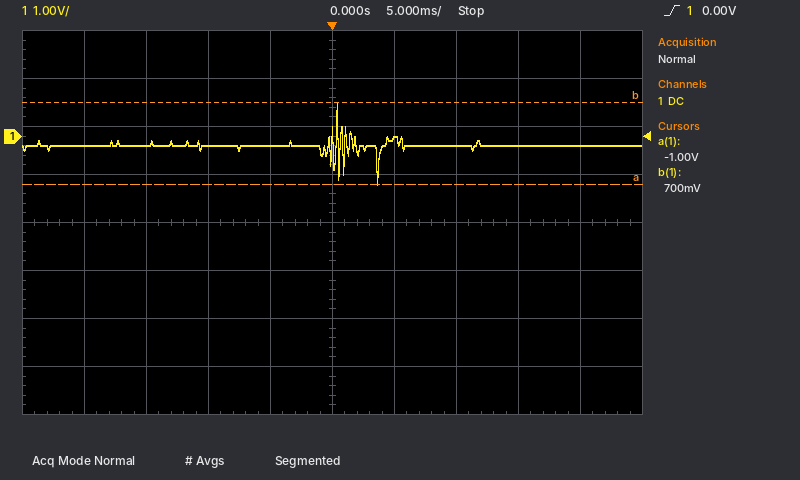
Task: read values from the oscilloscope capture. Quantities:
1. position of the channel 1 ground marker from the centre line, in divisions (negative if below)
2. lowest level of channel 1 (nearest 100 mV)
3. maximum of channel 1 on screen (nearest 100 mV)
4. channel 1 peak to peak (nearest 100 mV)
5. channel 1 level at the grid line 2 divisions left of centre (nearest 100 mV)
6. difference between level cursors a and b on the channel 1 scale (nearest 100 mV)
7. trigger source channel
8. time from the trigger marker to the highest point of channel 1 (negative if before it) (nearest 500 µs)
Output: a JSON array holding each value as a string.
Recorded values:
["+1.8 div", "-1.0 V", "700 mV", "1.7 V", "-200 mV", "1.7 V", "channel 1", "+500 µs"]
